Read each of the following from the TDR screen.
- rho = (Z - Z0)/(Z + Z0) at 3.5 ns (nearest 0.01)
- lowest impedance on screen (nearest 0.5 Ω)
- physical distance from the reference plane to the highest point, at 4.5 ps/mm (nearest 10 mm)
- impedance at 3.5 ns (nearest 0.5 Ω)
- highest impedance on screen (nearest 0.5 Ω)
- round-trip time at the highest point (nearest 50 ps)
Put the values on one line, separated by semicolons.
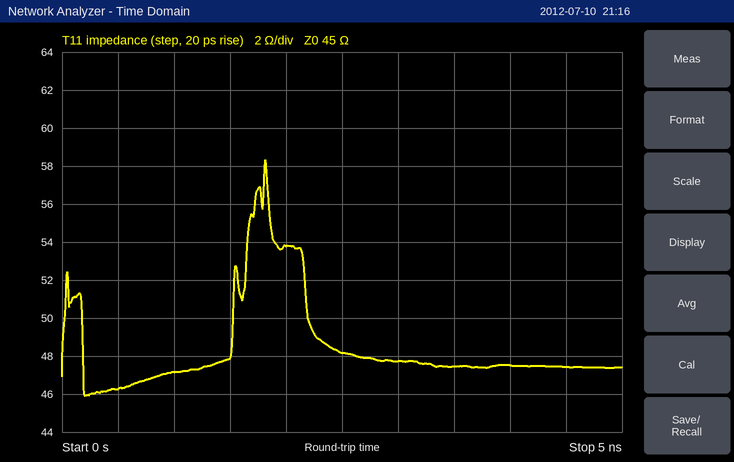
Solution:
+0.03; 46.0 Ω; 200 mm; 47.5 Ω; 58.5 Ω; 1.80 ns
